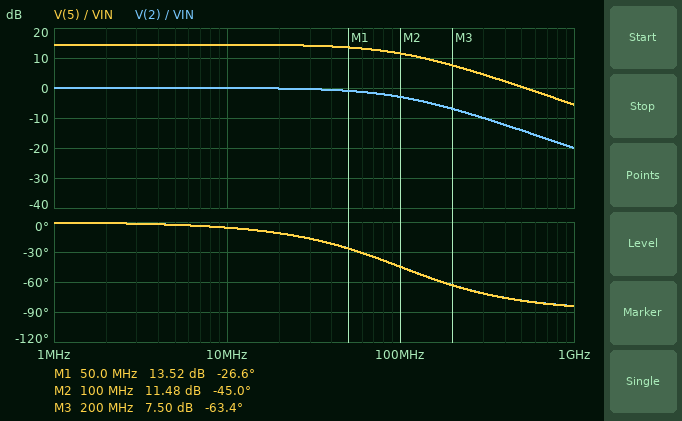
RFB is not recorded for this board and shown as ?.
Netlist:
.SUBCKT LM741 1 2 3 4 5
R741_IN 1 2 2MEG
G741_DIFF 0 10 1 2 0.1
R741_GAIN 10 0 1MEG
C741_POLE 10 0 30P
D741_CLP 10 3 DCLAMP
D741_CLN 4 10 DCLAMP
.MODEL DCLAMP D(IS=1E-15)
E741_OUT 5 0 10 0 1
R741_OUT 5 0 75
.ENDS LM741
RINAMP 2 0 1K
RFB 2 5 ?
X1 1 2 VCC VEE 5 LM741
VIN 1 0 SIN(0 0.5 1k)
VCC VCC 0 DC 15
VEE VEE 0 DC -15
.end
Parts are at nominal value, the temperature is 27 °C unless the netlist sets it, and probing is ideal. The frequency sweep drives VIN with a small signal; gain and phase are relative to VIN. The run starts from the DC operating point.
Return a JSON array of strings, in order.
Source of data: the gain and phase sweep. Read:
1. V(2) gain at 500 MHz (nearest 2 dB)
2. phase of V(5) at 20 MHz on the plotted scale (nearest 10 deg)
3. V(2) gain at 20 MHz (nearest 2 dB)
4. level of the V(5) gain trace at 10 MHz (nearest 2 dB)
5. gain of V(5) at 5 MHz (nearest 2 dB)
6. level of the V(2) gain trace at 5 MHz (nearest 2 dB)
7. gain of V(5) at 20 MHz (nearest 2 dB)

["-14 dB", "-10 deg", "0 dB", "14 dB", "14 dB", "0 dB", "14 dB"]
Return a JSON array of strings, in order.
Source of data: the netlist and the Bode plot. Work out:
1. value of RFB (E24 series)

["4.3 kΩ"]
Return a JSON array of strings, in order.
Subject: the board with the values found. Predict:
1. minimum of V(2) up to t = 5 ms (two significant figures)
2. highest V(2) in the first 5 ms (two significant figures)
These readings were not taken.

["-500 mV", "500 mV"]
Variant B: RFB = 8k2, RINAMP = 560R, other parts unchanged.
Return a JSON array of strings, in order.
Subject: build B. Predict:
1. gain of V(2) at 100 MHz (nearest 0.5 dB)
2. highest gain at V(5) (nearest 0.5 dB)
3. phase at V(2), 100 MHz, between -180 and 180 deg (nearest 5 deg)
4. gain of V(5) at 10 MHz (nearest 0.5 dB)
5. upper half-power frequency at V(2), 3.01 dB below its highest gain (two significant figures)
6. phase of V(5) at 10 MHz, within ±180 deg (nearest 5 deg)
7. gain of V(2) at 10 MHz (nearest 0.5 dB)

["-10.0 dB", "24.0 dB", "-70 deg", "23.5 dB", "34 MHz", "-15 deg", "-0.5 dB"]
